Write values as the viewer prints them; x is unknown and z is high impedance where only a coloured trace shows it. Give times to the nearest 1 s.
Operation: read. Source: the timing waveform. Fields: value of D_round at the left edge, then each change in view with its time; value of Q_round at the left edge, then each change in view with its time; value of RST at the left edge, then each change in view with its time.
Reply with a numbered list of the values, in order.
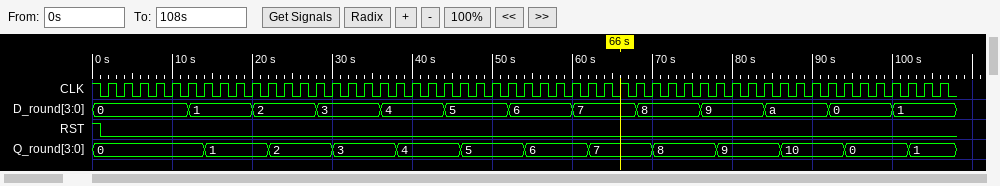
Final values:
1. 0, 1 at 12 s, 2 at 20 s, 3 at 28 s, 4 at 36 s, 5 at 44 s, 6 at 52 s, 7 at 60 s, 8 at 68 s, 9 at 76 s, a at 84 s, 0 at 92 s, 1 at 100 s
2. 0, 1 at 14 s, 2 at 22 s, 3 at 30 s, 4 at 38 s, 5 at 46 s, 6 at 54 s, 7 at 62 s, 8 at 70 s, 9 at 78 s, 10 at 86 s, 0 at 94 s, 1 at 102 s
3. 1, 0 at 1 s
